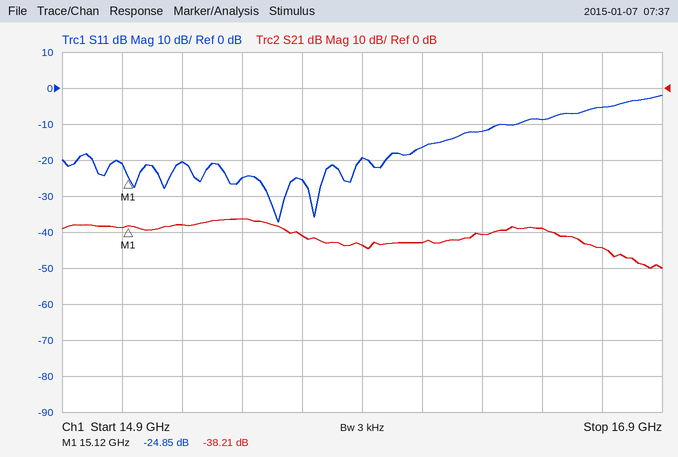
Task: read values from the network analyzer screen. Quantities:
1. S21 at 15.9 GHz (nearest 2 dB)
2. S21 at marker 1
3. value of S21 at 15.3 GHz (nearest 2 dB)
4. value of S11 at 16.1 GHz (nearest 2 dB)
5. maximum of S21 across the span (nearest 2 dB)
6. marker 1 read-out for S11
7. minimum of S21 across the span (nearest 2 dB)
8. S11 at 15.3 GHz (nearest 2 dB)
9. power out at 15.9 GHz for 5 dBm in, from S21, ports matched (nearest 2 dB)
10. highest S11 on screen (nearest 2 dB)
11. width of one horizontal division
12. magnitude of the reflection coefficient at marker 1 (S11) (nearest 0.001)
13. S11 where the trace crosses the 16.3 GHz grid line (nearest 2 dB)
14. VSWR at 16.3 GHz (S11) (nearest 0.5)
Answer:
-44 dB
-38.21 dB
-38 dB
-16 dB
-36 dB
-24.85 dB
-50 dB
-20 dB
-38 dBm
-2 dB
200 MHz
0.057
-12 dB
1.5
